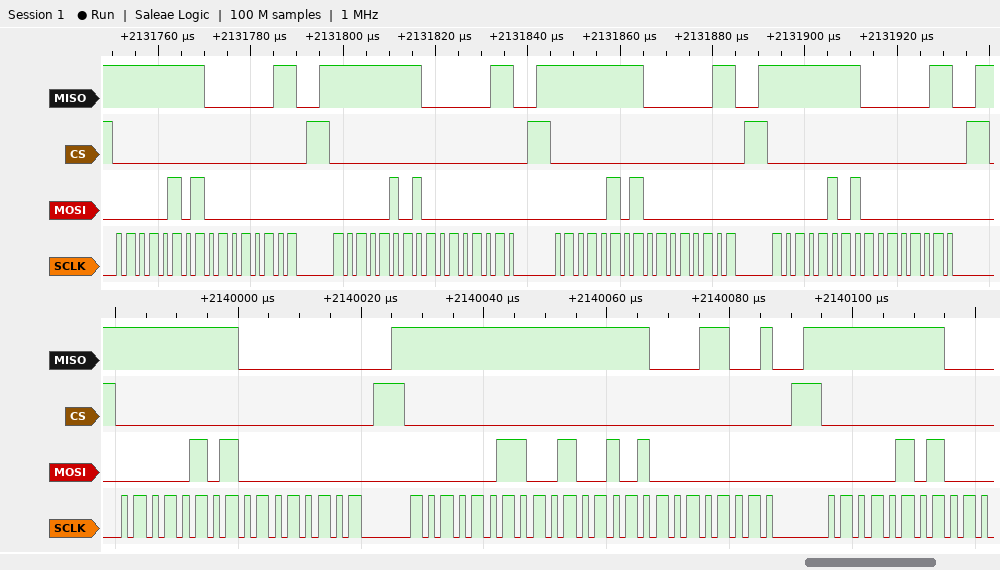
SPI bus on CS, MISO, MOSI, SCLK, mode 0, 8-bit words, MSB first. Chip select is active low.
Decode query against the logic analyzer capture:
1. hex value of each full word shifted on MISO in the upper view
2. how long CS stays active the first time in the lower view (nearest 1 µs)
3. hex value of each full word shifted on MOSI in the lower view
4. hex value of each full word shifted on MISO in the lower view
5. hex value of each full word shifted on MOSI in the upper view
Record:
FF, 03, FF, 03, FF, 03, FF, 03
42 µs
05, 00, 03, 25, 00, 05
FF, 00, FF, FF, 19, FF
05, 00, 05, 00, 05, 00, 05, 00
